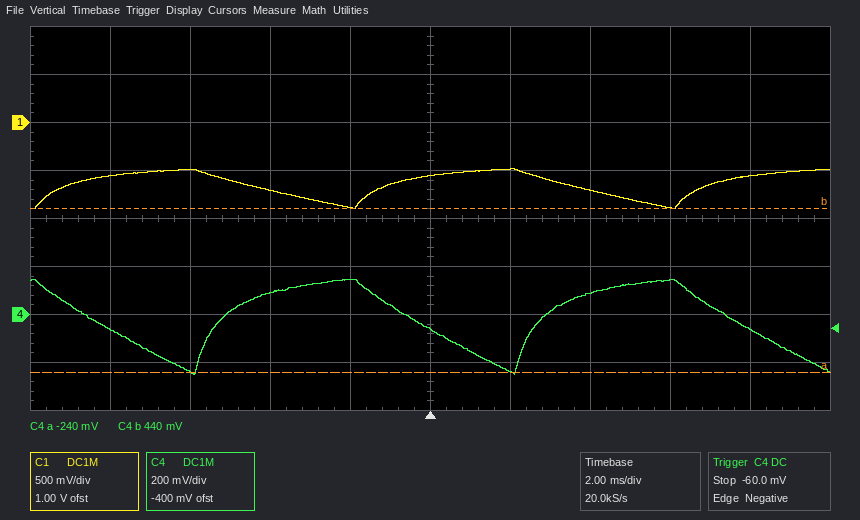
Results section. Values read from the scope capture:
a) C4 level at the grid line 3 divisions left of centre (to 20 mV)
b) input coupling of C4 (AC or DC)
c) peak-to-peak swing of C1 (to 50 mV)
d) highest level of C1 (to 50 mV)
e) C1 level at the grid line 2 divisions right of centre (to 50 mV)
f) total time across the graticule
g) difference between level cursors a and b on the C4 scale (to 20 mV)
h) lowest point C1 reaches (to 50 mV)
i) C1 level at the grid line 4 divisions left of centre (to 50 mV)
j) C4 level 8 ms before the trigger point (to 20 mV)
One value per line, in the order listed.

-240 mV
DC
400 mV
-500 mV
-700 mV
20 ms
680 mV
-900 mV
-550 mV
-60 mV
